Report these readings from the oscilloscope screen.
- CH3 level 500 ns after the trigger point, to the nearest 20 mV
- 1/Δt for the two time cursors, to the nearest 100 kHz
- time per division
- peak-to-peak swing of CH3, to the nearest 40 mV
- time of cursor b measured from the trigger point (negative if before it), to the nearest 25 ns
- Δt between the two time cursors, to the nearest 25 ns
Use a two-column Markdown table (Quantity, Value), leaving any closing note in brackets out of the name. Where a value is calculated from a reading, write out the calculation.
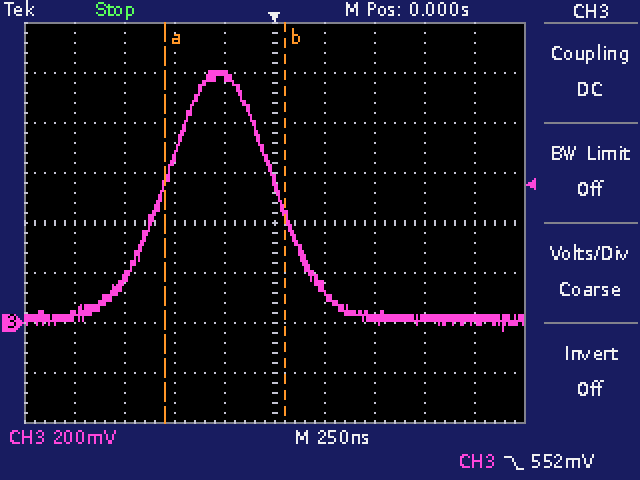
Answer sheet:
| Quantity | Value |
|---|---|
| CH3 level 500 ns after the trigger point, to the nearest 20 mV | 20 mV |
| 1/Δt for the two time cursors, to the nearest 100 kHz | 1 / 600 ns ≈ 1.7 MHz |
| time per division | 250 ns |
| peak-to-peak swing of CH3, to the nearest 40 mV | 1.04 V |
| time of cursor b measured from the trigger point (negative if before it), to the nearest 25 ns | +50 ns |
| Δt between the two time cursors, to the nearest 25 ns | 600 ns |
